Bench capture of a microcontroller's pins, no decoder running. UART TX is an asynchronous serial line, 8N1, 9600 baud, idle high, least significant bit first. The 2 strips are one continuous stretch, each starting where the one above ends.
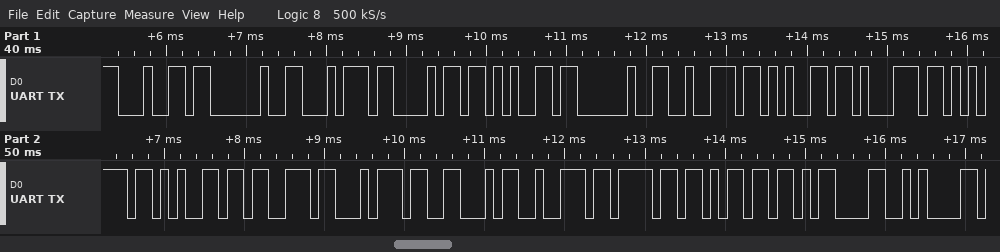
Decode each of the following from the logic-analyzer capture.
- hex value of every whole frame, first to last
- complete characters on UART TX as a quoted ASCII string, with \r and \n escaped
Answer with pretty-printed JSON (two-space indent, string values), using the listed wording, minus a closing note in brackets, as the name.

{
  "hex value of every whole frame, first to last": "64 20 74 68 65 20 72 65 71 75 65 73 74 46 72 6F 6D 0D 0A",
  "complete characters on UART TX as a quoted ASCII string, with \\r and \\n escaped": "\"d the requestFrom\\r\\n\""
}
